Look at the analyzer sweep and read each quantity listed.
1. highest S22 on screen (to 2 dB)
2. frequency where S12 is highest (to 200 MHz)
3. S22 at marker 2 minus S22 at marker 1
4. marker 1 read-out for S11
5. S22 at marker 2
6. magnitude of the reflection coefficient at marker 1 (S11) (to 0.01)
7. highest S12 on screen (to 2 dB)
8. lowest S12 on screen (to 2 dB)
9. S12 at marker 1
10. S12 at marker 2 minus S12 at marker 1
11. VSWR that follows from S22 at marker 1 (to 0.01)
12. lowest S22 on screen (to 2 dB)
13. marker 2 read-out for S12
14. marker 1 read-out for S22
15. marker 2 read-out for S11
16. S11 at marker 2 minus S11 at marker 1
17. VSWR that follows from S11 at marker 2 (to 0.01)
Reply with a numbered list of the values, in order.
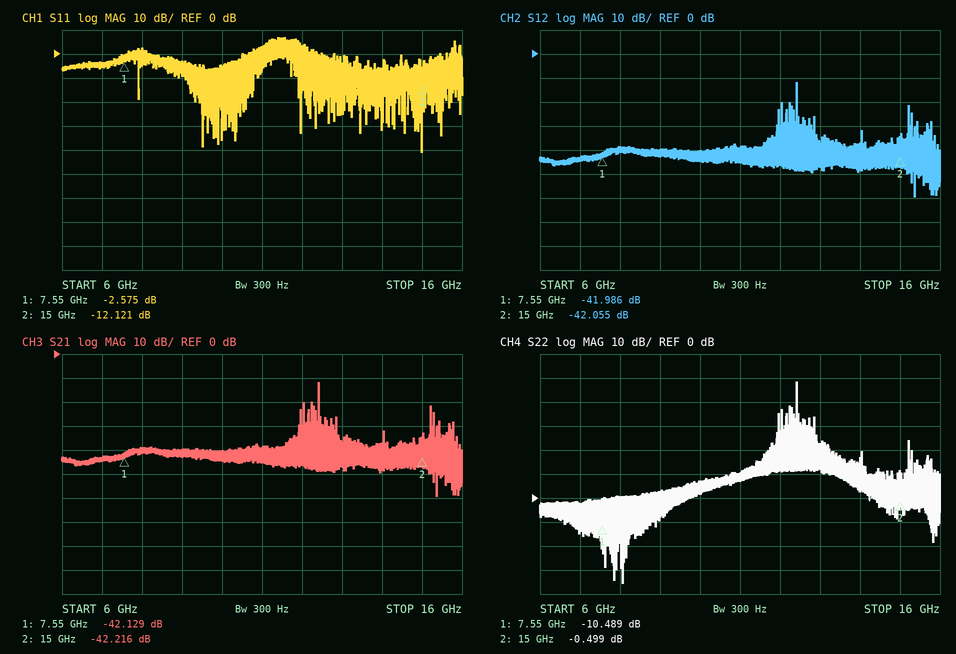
1. 48 dB
2. 12.4 GHz
3. 9.990 dB
4. -2.575 dB
5. -0.499 dB
6. 0.74
7. -12 dB
8. -60 dB
9. -41.986 dB
10. -0.069 dB
11. 1.85
12. -36 dB
13. -42.055 dB
14. -10.489 dB
15. -12.121 dB
16. -9.546 dB
17. 1.66
